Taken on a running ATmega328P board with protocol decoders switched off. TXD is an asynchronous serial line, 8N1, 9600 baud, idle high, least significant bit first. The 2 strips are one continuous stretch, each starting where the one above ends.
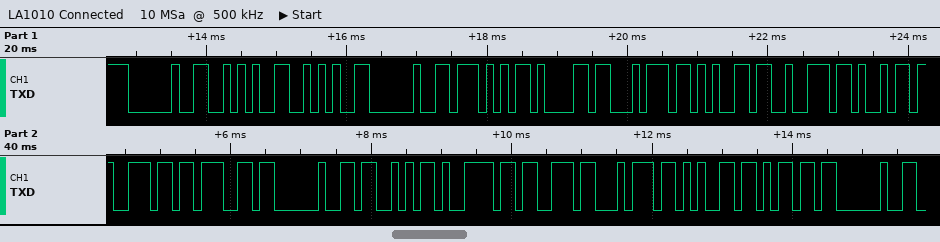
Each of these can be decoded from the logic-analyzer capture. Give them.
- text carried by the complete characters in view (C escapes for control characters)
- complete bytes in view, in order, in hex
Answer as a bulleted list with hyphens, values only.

- " ** Watering System "
- 20 2A 2A 20 57 61 74 65 72 69 6E 67 20 53 79 73 74 65 6D 20
